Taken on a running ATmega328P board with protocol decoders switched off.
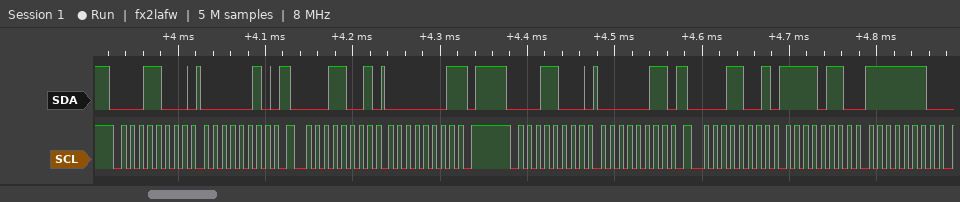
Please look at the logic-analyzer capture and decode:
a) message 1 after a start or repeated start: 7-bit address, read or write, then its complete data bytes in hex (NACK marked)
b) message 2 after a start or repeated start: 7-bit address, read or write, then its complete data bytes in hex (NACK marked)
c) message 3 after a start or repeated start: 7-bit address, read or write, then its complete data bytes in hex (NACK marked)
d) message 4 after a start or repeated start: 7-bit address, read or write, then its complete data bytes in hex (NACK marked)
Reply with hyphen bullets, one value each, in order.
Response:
- 0x0C write: 02
- 0x0C read: 01 NACK
- 0x0C write: 03
- 0x0C read: F6 FE
